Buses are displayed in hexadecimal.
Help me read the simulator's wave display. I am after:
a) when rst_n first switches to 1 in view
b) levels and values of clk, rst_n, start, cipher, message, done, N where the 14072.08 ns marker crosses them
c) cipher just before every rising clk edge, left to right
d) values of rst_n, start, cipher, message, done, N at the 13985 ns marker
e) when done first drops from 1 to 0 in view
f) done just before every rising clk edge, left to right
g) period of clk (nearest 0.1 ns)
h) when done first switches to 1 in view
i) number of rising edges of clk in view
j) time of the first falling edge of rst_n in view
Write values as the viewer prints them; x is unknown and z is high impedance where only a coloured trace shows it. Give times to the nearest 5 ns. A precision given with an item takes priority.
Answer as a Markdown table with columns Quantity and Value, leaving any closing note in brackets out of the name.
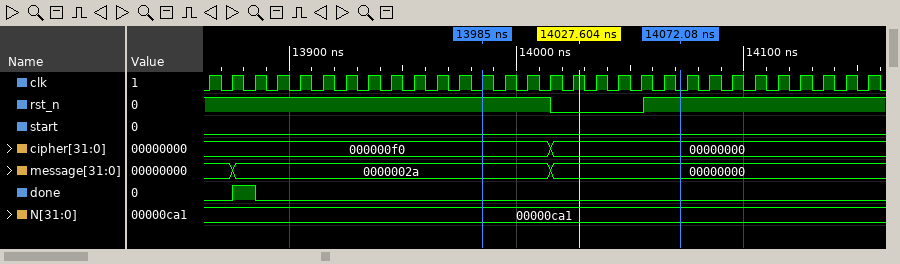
| Quantity | Value |
|---|---|
| when rst_n first switches to 1 in view | 14055 ns |
| levels and values of clk, rst_n, start, cipher, message, done, N where the 14072.08 ns marker crosses them | clk=0, rst_n=1, start=0, cipher=00000000, message=00000000, done=0, N=00000ca1 |
| cipher just before every rising clk edge, left to right | 000000f0, 000000f0, 000000f0, 000000f0, 000000f0, 000000f0, 000000f0, 000000f0, 000000f0, 000000f0, 000000f0, 000000f0, 000000f0, 000000f0, 000000f0, 000000f0, 00000000, 00000000, 00000000, 00000000, 00000000, 00000000, 00000000, 00000000, 00000000, 00000000, 00000000, 00000000, 00000000, 00000000 |
| values of rst_n, start, cipher, message, done, N at the 13985 ns marker | rst_n=1, start=0, cipher=000000f0, message=0000002a, done=0, N=00000ca1 |
| when done first drops from 1 to 0 in view | 13885 ns |
| done just before every rising clk edge, left to right | 0 0 1 0 0 0 0 0 0 0 0 0 0 0 0 0 0 0 0 0 0 0 0 0 0 0 0 0 0 0 |
| period of clk | 10 ns |
| when done first switches to 1 in view | 13875 ns |
| number of rising edges of clk in view | 30 |
| time of the first falling edge of rst_n in view | 14015 ns |
